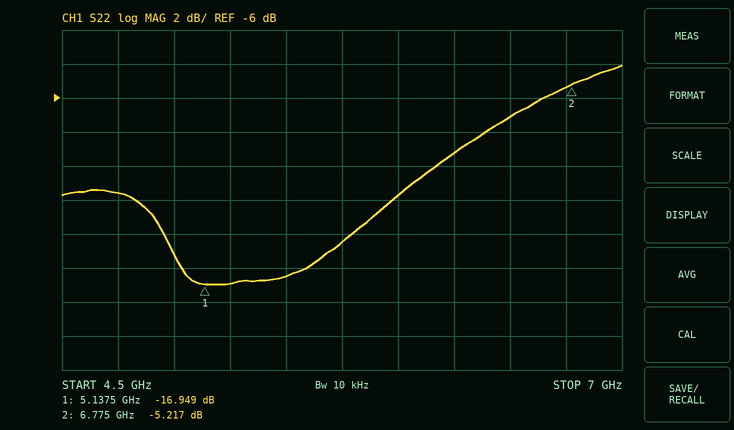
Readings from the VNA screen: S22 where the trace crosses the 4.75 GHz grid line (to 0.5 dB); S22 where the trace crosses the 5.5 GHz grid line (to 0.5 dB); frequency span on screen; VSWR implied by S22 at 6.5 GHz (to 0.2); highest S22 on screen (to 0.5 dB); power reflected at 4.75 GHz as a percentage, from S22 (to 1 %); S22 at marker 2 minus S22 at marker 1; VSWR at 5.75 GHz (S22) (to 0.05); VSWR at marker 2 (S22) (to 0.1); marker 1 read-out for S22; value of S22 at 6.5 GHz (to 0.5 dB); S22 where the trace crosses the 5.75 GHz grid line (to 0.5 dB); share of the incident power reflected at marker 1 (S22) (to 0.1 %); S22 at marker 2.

-11.5 dB
-16.5 dB
2.5 GHz
2.6
-4.0 dB
7 %
11.732 dB
1.45
3.4
-16.949 dB
-7.0 dB
-14.5 dB
2.0 %
-5.217 dB
